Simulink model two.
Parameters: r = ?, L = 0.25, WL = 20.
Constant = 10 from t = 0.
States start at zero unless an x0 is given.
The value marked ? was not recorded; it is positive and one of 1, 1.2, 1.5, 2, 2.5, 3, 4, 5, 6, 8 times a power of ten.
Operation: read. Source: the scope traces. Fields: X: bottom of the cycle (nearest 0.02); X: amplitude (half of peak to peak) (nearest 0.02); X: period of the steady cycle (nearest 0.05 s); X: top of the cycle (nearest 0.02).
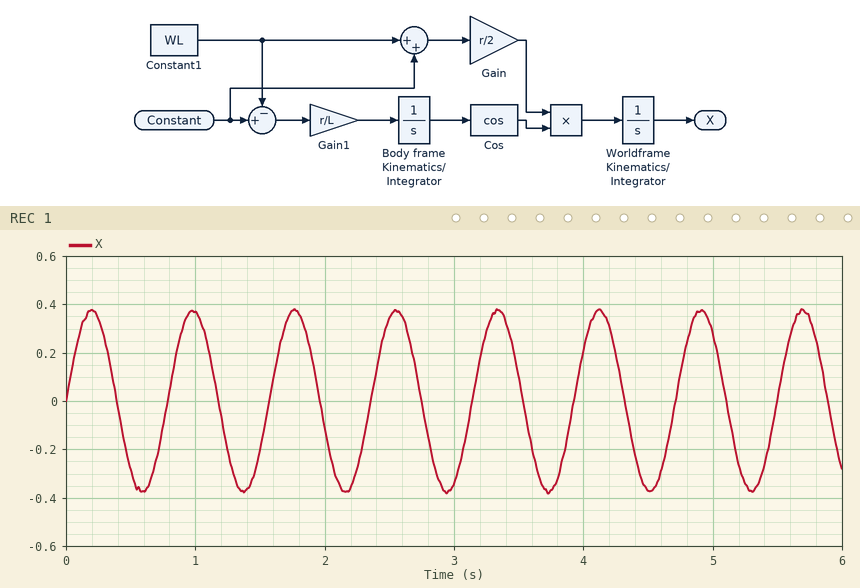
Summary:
-0.38
0.38
0.80 s
0.38
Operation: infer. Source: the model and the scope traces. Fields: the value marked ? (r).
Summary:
0.2
